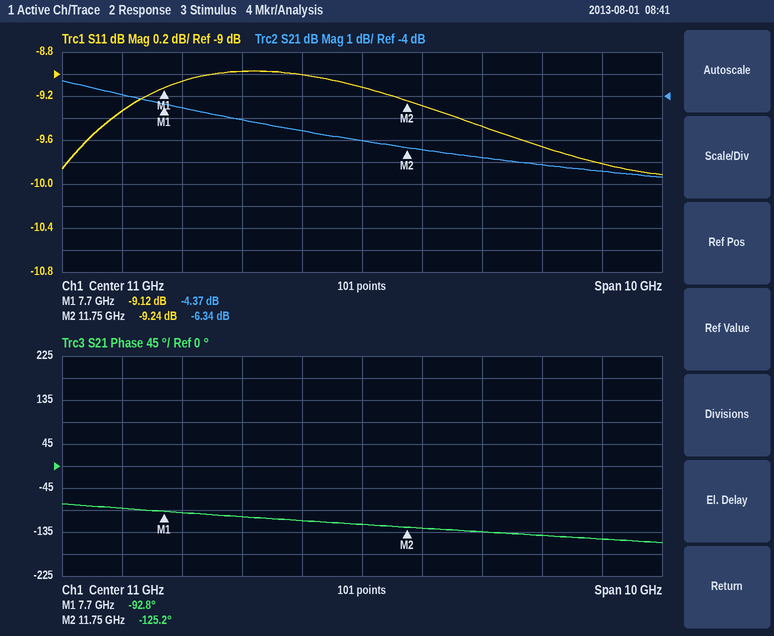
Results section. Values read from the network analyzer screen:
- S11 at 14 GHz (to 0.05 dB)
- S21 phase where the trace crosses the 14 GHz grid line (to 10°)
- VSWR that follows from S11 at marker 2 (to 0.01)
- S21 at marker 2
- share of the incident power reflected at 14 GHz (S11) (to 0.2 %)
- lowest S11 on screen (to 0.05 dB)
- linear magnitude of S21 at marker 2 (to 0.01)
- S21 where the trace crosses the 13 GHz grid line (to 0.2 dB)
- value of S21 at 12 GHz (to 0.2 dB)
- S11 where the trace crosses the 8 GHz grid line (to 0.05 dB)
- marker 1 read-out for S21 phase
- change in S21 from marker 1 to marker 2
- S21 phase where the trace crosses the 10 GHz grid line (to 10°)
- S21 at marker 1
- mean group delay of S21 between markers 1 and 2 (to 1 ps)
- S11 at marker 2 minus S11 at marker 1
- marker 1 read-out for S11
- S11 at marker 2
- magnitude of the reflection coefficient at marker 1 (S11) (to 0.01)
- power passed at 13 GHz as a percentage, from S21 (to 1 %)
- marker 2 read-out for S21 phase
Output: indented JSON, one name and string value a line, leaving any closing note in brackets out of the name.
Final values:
{
  "S11 at 14 GHz": "-9.65 dB",
  "S21 phase where the trace crosses the 14 GHz grid line": "-140°",
  "VSWR that follows from S11 at marker 2": "2.05",
  "S21 at marker 2": "-6.34 dB",
  "share of the incident power reflected at 14 GHz (S11)": "10.8 %",
  "lowest S11 on screen": "-9.90 dB",
  "linear magnitude of S21 at marker 2": "0.48",
  "S21 where the trace crosses the 13 GHz grid line": "-6.8 dB",
  "value of S21 at 12 GHz": "-6.4 dB",
  "S11 where the trace crosses the 8 GHz grid line": "-9.05 dB",
  "marker 1 read-out for S21 phase": "-92.8°",
  "change in S21 from marker 1 to marker 2": "-1.97 dB",
  "S21 phase where the trace crosses the 10 GHz grid line": "-110°",
  "S21 at marker 1": "-4.37 dB",
  "mean group delay of S21 between markers 1 and 2": "22 ps",
  "S11 at marker 2 minus S11 at marker 1": "-0.12 dB",
  "marker 1 read-out for S11": "-9.12 dB",
  "S11 at marker 2": "-9.24 dB",
  "magnitude of the reflection coefficient at marker 1 (S11)": "0.35",
  "power passed at 13 GHz as a percentage, from S21": "21 %",
  "marker 2 read-out for S21 phase": "-125.2°"
}
